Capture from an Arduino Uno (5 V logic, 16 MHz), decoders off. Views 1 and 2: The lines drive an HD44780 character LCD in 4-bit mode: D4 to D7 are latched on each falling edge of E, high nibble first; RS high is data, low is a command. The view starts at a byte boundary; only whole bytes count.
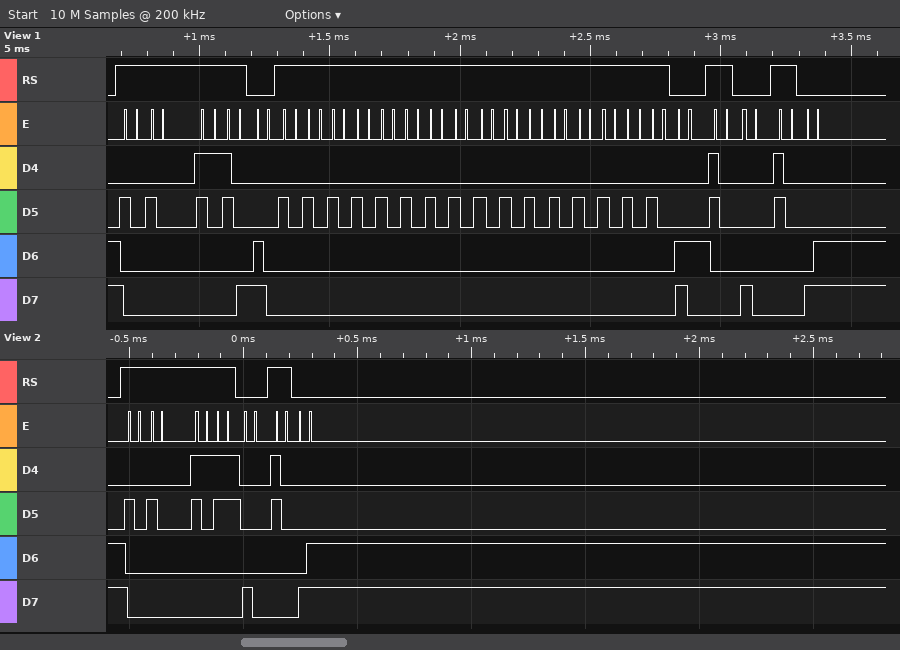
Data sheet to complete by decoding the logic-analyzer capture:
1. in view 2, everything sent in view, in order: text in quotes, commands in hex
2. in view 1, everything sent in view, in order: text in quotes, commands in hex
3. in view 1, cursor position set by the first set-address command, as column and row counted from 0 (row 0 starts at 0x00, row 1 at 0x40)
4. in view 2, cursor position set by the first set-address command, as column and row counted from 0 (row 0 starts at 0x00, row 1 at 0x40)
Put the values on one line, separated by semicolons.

"  13" 0x80 "0" 0x8C; "  18" 0xC0 "                " 0xC4 "0" 0x80 "0" 0x8C; column 0, row 1; column 0, row 0
